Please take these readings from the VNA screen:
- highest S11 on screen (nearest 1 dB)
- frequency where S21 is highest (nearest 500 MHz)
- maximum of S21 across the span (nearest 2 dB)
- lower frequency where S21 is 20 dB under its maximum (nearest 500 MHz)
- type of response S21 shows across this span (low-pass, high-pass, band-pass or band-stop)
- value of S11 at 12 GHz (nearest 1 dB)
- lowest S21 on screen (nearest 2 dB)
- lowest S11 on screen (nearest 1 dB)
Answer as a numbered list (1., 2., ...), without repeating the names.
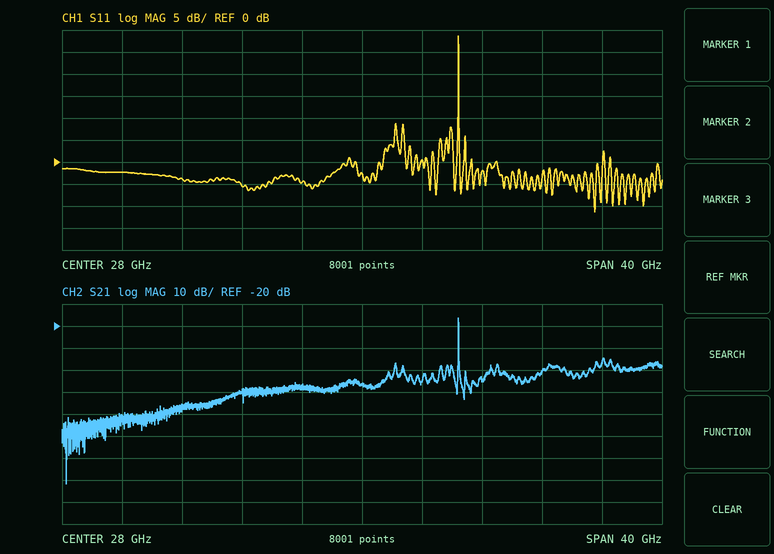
1. 29 dB
2. 34.5 GHz
3. -16 dB
4. 34.5 GHz
5. band-pass
6. -2 dB
7. -92 dB
8. -11 dB
